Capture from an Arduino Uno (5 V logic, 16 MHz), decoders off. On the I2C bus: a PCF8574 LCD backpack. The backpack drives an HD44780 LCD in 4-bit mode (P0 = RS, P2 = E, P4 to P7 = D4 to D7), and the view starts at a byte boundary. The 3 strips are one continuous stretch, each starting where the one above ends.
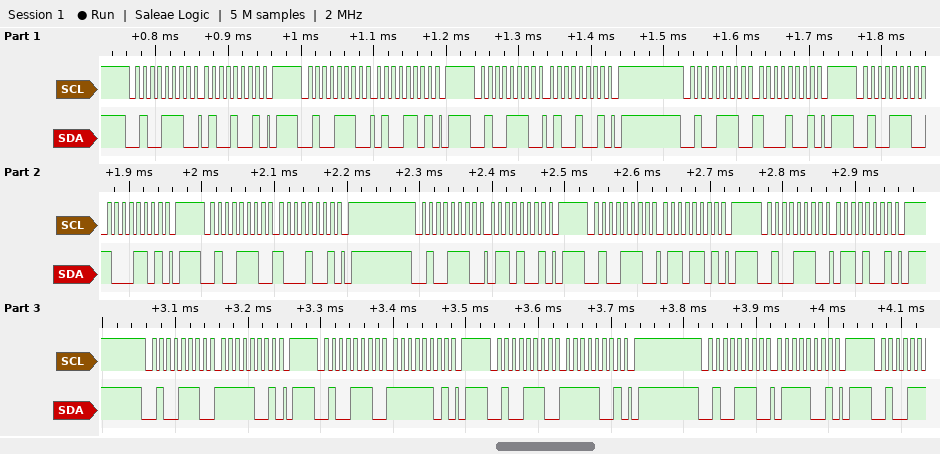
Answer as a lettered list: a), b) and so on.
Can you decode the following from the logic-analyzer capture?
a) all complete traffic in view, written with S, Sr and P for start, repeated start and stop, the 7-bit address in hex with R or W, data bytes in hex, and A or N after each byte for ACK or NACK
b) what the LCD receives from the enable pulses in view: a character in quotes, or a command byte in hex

a) S 27W A 49 A P S 27W A 4D A P S 27W A 49 A P S 27W A 89 A P S 27W A 8D A P S 27W A 89 A P S 27W A 69 A P S 27W A 6D A P S 27W A 69 A P S 27W A F9 A P S 27W A FD A P S 27W A F9 A P S 27W A 79 A P
b) 'H' 'o'
